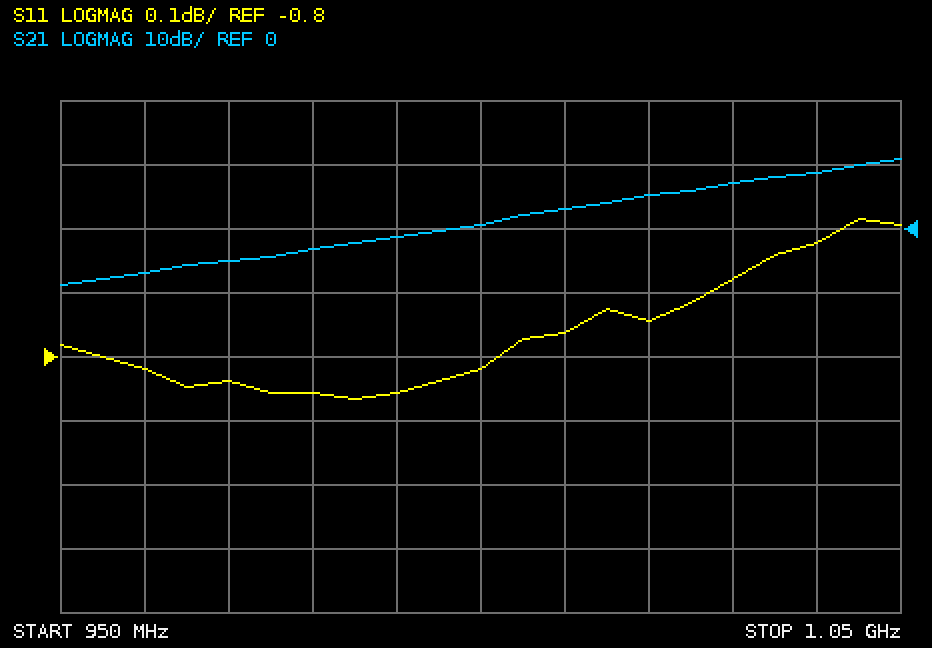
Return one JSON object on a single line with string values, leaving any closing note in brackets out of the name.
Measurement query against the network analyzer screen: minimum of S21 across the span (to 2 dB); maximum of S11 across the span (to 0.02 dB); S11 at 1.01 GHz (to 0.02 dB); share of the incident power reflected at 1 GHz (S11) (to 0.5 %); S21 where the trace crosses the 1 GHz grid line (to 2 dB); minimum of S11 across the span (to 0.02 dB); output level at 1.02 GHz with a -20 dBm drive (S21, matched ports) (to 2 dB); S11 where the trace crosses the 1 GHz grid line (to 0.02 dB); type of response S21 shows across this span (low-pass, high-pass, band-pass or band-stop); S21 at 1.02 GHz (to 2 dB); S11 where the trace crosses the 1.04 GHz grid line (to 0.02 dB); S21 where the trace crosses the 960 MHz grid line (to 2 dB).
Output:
{"minimum of S21 across the span": "-8 dB", "maximum of S11 across the span": "-0.58 dB", "S11 at 1.01 GHz": "-0.76 dB", "share of the incident power reflected at 1 GHz (S11)": "83.0 %", "S21 where the trace crosses the 1 GHz grid line": "0 dB", "minimum of S11 across the span": "-0.86 dB", "output level at 1.02 GHz with a -20 dBm drive (S21, matched ports)": "-14 dBm", "S11 where the trace crosses the 1 GHz grid line": "-0.82 dB", "type of response S21 shows across this span": "high-pass", "S21 at 1.02 GHz": "6 dB", "S11 where the trace crosses the 1.04 GHz grid line": "-0.62 dB", "S21 where the trace crosses the 960 MHz grid line": "-6 dB"}
